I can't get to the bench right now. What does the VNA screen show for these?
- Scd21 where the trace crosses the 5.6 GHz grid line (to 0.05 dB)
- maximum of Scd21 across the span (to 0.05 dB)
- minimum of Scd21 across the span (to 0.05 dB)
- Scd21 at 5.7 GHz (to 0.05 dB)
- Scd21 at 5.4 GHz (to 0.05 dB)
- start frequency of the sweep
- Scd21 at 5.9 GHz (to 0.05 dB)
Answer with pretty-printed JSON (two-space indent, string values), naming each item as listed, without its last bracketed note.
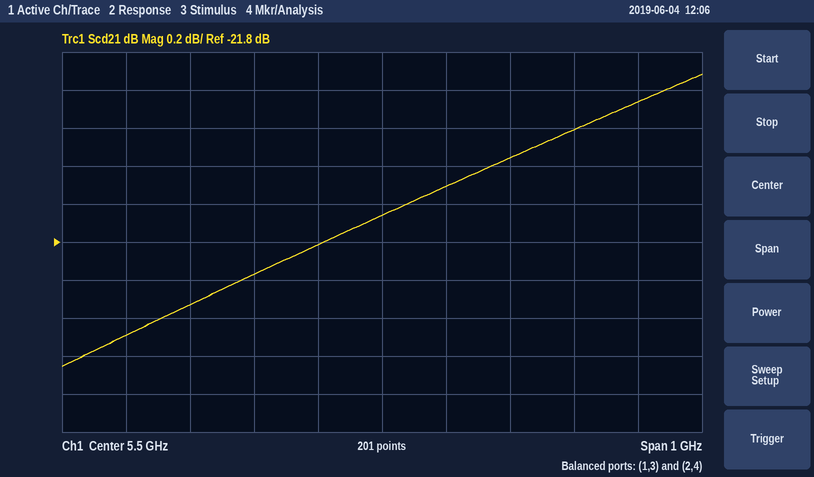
{
  "Scd21 where the trace crosses the 5.6 GHz grid line": "-21.50 dB",
  "maximum of Scd21 across the span": "-20.90 dB",
  "minimum of Scd21 across the span": "-22.45 dB",
  "Scd21 at 5.7 GHz": "-21.35 dB",
  "Scd21 at 5.4 GHz": "-21.80 dB",
  "start frequency of the sweep": "5 GHz",
  "Scd21 at 5.9 GHz": "-21.05 dB"
}
